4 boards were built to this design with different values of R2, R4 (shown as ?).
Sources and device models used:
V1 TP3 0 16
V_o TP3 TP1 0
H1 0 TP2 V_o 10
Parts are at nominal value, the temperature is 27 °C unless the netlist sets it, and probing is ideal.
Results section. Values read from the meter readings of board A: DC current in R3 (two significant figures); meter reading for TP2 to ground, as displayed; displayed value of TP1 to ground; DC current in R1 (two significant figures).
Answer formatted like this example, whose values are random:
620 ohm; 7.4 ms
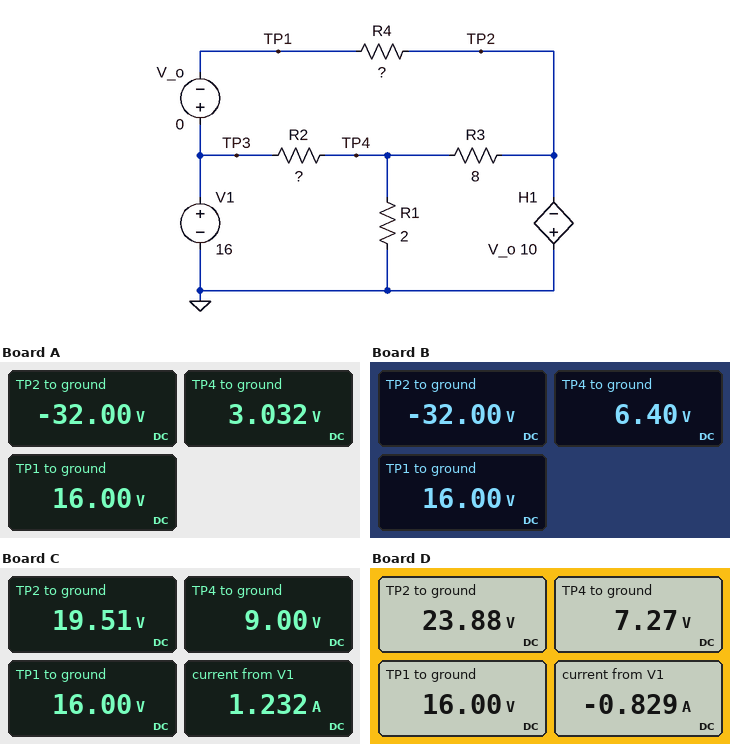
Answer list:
4.4 A; -32.00 V; 16.00 V; 1.5 A
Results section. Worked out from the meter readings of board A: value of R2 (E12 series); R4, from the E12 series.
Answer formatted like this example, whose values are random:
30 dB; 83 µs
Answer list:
2.2 Ω; 15 Ω
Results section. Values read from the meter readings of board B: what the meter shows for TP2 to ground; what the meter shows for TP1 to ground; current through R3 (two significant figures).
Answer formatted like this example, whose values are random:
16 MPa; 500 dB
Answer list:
-32.00 V; 16.00 V; 4.8 A
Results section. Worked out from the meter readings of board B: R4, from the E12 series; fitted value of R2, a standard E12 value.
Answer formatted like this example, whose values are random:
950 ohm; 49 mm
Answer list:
15 Ω; 1.2 Ω
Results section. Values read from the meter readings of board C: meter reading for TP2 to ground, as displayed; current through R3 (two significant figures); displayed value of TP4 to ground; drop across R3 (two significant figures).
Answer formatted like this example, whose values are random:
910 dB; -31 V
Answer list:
19.51 V; 1.3 A; 9.00 V; 11 V
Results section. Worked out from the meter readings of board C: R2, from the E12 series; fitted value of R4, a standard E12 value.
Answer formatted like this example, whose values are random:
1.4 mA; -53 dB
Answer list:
2.2 Ω; 1.8 Ω
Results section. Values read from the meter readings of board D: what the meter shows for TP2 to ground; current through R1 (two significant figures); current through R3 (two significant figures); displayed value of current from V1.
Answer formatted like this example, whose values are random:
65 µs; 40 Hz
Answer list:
23.88 V; 3.6 A; 2.1 A; -0.829 A
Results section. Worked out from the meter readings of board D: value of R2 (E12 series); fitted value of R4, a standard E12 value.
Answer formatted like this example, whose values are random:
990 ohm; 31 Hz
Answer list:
5.6 Ω; 3.3 Ω
